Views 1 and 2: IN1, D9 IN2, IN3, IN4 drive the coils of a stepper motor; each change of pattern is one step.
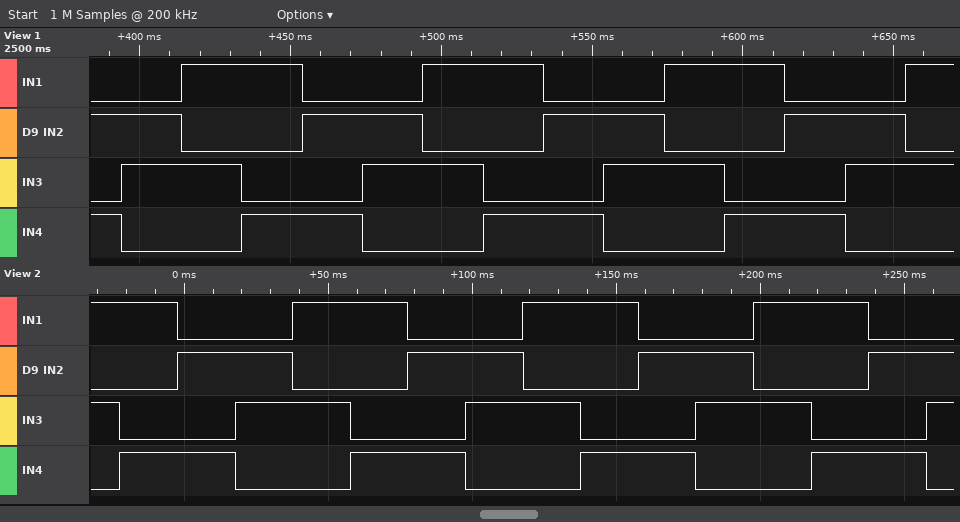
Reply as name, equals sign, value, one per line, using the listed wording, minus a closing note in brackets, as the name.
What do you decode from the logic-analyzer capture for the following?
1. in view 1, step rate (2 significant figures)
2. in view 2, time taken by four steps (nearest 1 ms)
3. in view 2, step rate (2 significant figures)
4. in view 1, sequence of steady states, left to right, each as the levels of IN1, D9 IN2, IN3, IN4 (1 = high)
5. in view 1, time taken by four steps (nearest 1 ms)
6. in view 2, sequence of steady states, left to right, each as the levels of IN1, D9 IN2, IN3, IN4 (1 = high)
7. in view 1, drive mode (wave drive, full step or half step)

in view 1, step rate = 50 steps/s
in view 2, time taken by four steps = 80 ms
in view 2, step rate = 50 steps/s
in view 1, sequence of steady states, left to right, each as the levels of IN1, D9 IN2, IN3, IN4 = 0101 0110 1010 1001 0101 0110 1010 1001 0101 0110 1010 1001 0101 0110 1010
in view 1, time taken by four steps = 80 ms
in view 2, sequence of steady states, left to right, each as the levels of IN1, D9 IN2, IN3, IN4 = 1010 1001 0101 0110 1010 1001 0101 0110 1010 1001 0101 0110 1010 1001 0101 0110
in view 1, drive mode = full step
